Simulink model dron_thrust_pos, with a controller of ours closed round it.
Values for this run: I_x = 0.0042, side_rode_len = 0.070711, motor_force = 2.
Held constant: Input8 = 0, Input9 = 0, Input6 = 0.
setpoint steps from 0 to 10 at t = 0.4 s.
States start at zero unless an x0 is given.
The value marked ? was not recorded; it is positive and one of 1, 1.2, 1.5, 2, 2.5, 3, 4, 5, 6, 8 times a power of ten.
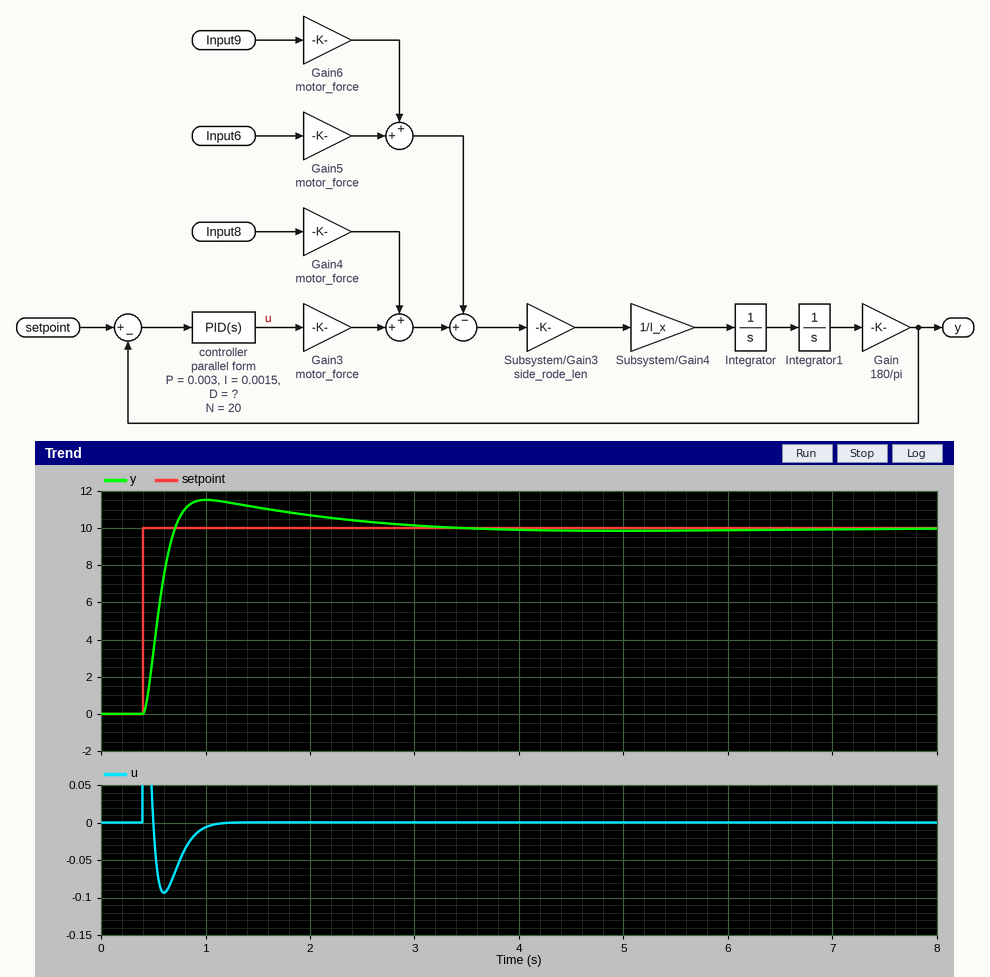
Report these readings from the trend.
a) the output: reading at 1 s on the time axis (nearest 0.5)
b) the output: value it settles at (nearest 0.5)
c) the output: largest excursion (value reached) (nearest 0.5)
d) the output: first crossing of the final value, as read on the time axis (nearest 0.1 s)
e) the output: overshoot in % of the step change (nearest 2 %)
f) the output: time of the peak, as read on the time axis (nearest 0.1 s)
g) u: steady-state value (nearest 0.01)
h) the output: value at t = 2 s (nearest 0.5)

11.5
10.0
11.5
0.7 s
16 %
1.0 s
0.00
10.5
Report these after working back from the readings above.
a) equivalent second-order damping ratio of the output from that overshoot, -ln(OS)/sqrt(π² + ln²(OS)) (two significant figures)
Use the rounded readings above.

0.50
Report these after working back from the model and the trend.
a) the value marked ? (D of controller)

0.003
